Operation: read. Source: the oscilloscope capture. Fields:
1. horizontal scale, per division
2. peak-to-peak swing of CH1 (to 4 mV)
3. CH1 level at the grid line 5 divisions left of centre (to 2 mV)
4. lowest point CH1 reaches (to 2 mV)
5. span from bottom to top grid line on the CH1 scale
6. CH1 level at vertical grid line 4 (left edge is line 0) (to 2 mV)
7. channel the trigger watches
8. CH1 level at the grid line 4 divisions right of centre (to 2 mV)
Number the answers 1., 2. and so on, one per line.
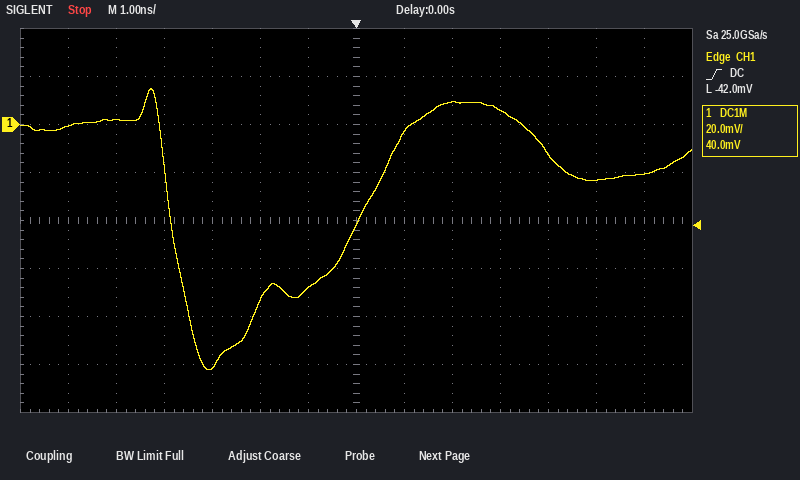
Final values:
1. 1 ns
2. 116 mV
3. 2 mV
4. -102 mV
5. 160 mV
6. -102 mV
7. CH1
8. -12 mV
